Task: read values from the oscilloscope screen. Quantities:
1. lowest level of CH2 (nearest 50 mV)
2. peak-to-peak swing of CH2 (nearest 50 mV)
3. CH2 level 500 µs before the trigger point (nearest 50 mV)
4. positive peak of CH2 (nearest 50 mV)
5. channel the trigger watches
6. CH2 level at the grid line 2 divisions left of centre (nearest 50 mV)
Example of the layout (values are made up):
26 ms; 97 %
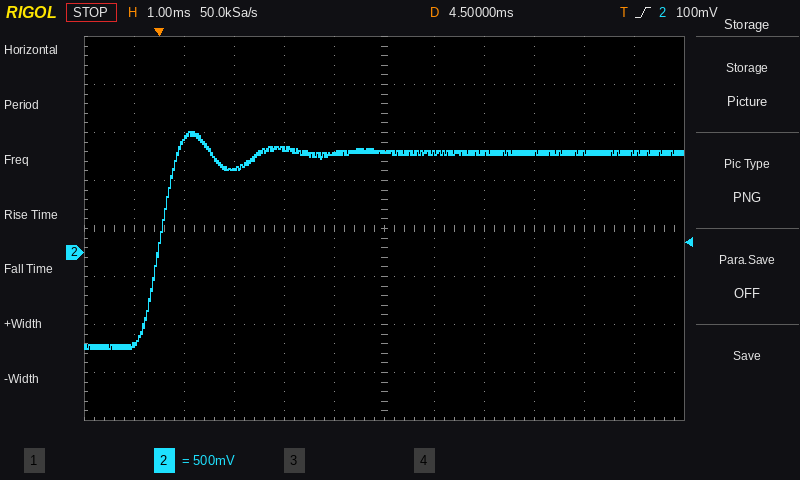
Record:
-1.00 V; 2.25 V; -950 mV; 1.25 V; CH2; 1.10 V
